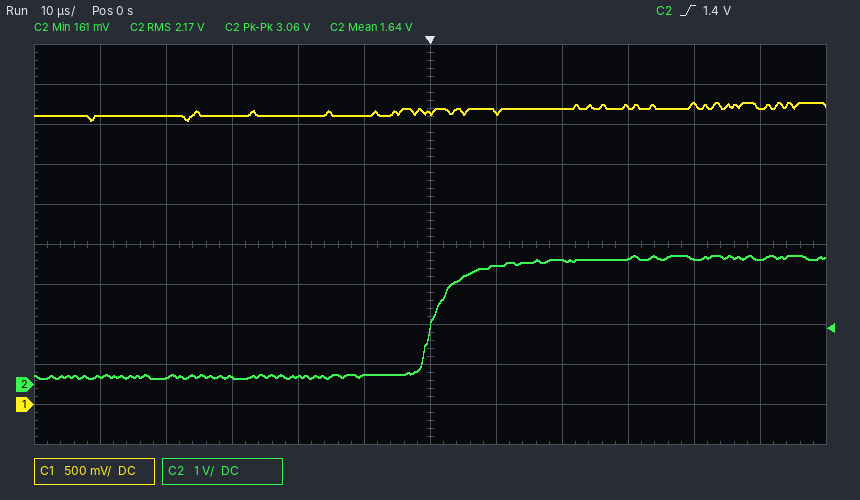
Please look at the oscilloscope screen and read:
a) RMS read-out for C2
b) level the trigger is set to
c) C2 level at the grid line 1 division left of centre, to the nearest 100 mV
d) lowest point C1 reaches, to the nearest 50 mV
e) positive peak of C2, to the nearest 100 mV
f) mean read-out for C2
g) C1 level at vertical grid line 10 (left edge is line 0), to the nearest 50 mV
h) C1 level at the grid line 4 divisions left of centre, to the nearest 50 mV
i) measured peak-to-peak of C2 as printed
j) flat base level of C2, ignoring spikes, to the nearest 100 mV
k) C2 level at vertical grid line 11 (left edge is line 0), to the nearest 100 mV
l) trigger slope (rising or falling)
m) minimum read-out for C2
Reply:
2.17 V
1.4 V
200 mV
3.55 V
3.2 V
1.64 V
3.75 V
3.60 V
3.06 V
200 mV
3.1 V
rising
161 mV
